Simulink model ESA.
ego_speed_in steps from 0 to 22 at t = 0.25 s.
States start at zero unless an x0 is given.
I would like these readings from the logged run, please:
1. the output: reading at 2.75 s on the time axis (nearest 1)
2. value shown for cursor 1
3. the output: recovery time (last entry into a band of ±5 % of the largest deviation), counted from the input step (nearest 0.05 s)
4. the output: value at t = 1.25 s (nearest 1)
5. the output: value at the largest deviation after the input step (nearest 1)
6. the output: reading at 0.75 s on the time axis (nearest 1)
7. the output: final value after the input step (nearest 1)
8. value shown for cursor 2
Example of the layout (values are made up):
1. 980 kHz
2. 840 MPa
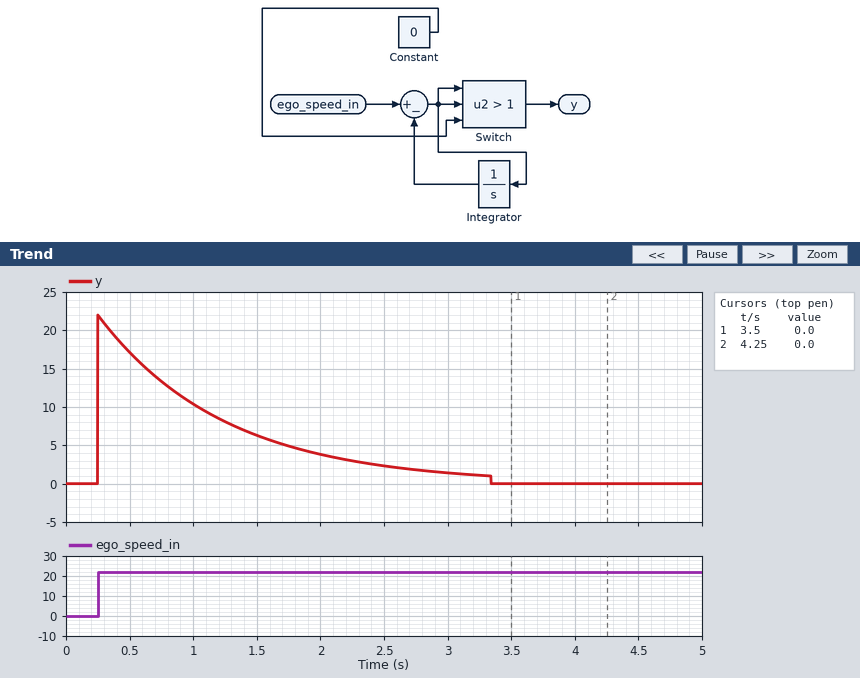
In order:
1. 2
2. 0.0
3. 3.00 s
4. 8
5. 22
6. 13
7. 0
8. 0.0
